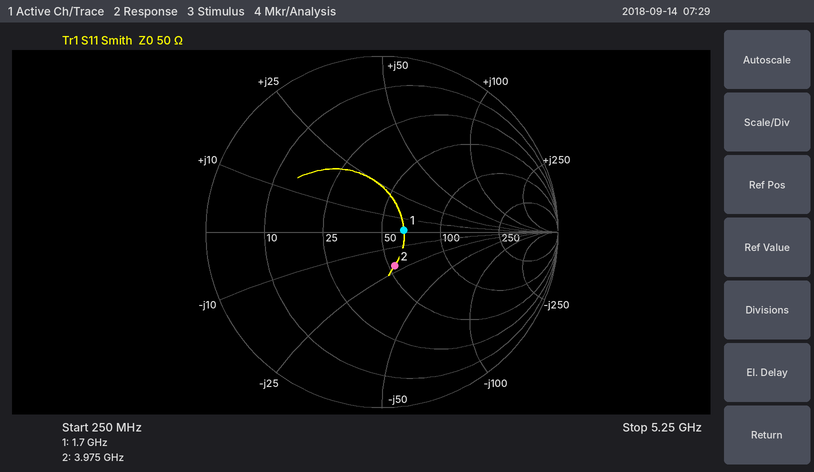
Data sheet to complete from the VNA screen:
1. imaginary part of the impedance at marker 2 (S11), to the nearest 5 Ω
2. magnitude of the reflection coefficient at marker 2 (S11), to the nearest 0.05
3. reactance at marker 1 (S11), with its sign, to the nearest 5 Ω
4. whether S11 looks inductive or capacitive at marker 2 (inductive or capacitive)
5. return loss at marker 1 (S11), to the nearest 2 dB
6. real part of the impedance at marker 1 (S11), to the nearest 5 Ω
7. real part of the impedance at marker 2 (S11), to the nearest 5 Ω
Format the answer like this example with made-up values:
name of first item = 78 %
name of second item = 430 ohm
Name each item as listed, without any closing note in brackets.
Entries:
imaginary part of the impedance at marker 2 (S11), to the nearest 5 Ω = -20 Ω
magnitude of the reflection coefficient at marker 2 (S11), to the nearest 0.05 = 0.20
reactance at marker 1 (S11), with its sign, to the nearest 5 Ω = 0 Ω
whether S11 looks inductive or capacitive at marker 2 = capacitive
return loss at marker 1 (S11), to the nearest 2 dB = 18 dB
real part of the impedance at marker 1 (S11), to the nearest 5 Ω = 65 Ω
real part of the impedance at marker 2 (S11), to the nearest 5 Ω = 55 Ω
